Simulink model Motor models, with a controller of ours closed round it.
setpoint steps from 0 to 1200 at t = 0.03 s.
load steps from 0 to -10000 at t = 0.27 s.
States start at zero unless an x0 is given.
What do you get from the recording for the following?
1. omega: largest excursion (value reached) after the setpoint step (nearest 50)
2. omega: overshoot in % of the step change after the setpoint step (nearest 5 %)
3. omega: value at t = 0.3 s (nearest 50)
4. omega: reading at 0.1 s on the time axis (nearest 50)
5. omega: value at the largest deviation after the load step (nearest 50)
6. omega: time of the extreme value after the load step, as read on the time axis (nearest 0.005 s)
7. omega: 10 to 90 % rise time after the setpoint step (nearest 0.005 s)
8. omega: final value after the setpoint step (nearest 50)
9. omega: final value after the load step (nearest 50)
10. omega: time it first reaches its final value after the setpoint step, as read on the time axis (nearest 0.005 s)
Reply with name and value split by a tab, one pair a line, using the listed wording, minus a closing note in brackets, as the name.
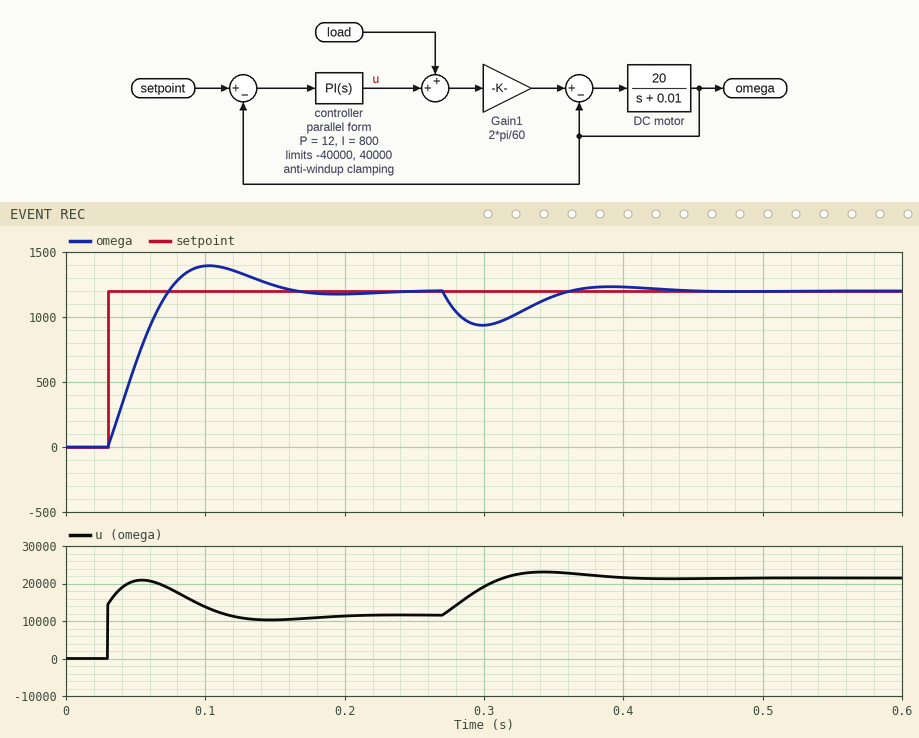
omega: largest excursion (value reached) after the setpoint step	1400
omega: overshoot in % of the step change after the setpoint step	15 %
omega: value at t = 0.3 s	950
omega: reading at 0.1 s on the time axis	1400
omega: value at the largest deviation after the load step	950
omega: time of the extreme value after the load step, as read on the time axis	0.300 s
omega: 10 to 90 % rise time after the setpoint step	0.035 s
omega: final value after the setpoint step	1200
omega: final value after the load step	1200
omega: time it first reaches its final value after the setpoint step, as read on the time axis	0.075 s
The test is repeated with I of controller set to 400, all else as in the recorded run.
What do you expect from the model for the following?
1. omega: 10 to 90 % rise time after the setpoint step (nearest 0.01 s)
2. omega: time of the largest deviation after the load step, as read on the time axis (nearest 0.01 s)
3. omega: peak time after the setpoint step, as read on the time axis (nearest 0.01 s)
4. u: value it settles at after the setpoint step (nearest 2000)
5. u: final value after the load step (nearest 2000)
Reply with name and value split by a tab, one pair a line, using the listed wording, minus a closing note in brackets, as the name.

omega: 10 to 90 % rise time after the setpoint step	0.05 s
omega: time of the largest deviation after the load step, as read on the time axis	0.31 s
omega: peak time after the setpoint step, as read on the time axis	0.15 s
u: value it settles at after the setpoint step	12000
u: final value after the load step	22000
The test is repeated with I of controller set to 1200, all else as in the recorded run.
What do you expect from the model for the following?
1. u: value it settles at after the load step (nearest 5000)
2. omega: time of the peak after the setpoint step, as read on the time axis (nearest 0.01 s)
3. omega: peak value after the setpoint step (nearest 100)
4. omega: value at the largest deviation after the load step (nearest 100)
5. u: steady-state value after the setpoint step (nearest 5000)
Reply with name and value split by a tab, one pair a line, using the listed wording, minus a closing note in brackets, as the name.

u: value it settles at after the load step	20000
omega: time of the peak after the setpoint step, as read on the time axis	0.09 s
omega: peak value after the setpoint step	1500
omega: value at the largest deviation after the load step	1000
u: steady-state value after the setpoint step	10000
